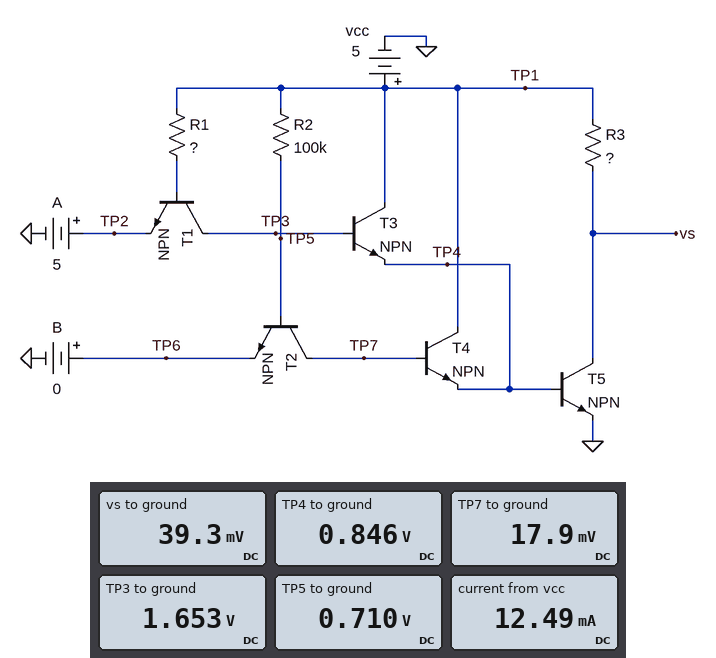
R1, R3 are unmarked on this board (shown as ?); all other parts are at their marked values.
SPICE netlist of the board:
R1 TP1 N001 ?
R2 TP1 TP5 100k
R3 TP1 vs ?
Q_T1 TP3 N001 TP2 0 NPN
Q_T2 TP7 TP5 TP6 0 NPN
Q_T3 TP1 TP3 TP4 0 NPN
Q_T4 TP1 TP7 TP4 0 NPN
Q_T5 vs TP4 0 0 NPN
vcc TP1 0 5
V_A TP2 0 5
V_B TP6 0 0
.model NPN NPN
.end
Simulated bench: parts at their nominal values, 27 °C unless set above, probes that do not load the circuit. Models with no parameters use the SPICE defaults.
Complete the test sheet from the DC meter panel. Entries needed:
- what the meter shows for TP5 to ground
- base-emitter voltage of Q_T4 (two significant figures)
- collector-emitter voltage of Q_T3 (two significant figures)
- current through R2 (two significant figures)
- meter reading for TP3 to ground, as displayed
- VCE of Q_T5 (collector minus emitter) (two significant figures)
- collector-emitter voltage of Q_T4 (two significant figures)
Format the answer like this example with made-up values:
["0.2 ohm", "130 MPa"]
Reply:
["0.710 V", "-830 mV", "4.2 V", "43 µA", "1.653 V", "39 mV", "4.2 V"]
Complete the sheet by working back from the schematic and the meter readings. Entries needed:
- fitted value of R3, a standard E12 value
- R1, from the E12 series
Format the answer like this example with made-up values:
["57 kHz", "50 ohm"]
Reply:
["560 Ω", "150 kΩ"]
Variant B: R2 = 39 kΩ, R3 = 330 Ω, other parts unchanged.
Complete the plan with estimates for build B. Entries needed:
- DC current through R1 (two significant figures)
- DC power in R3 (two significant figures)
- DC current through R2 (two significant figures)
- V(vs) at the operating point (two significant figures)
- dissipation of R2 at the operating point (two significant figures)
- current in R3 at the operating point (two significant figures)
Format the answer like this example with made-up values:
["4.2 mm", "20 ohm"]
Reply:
["18 µA", "74 mW", "110 µA", "48 mV", "470 µW", "15 mA"]
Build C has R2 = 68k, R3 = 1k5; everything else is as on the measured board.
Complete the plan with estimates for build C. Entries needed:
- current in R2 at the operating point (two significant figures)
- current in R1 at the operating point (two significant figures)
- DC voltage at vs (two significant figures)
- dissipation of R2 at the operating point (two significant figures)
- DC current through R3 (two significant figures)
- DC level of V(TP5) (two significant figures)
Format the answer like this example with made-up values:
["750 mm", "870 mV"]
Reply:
["63 µA", "18 µA", "28 mV", "270 µW", "3.3 mA", "720 mV"]
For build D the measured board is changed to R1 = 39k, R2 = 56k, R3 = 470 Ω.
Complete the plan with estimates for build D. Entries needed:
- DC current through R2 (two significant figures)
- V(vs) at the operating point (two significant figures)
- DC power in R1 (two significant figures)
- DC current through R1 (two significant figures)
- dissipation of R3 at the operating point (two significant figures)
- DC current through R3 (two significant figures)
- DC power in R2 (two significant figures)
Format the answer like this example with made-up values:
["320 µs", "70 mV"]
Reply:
["76 µA", "27 mV", "170 µW", "66 µA", "53 mW", "11 mA", "330 µW"]
